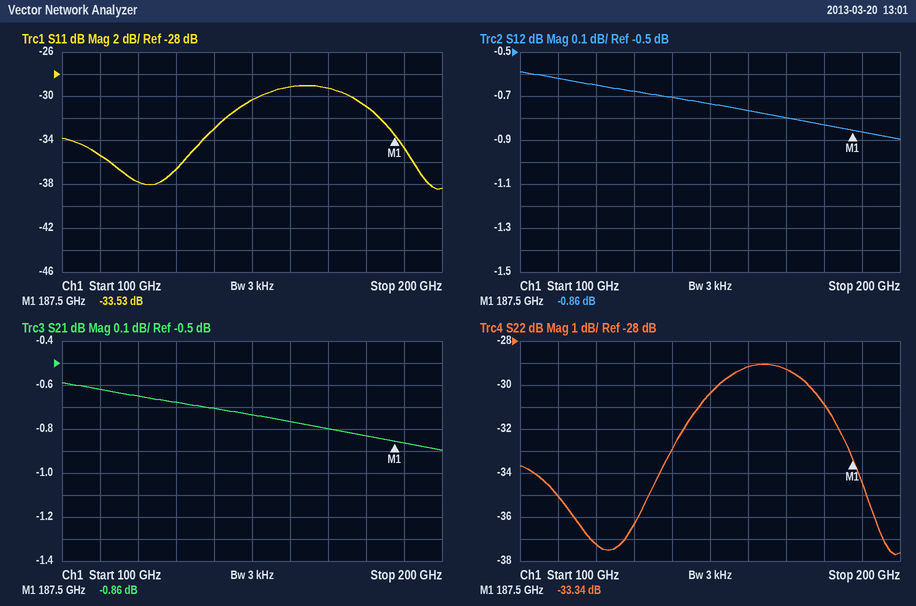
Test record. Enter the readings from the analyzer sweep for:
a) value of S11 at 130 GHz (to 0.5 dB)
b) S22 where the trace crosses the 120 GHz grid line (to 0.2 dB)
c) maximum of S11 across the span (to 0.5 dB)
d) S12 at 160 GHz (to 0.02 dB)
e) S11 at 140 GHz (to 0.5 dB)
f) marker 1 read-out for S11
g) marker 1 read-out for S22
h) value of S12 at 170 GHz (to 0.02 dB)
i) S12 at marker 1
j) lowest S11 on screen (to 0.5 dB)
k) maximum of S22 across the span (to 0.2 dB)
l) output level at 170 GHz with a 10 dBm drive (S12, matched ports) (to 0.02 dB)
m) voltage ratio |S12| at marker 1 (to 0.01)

-36.5 dB
-37.2 dB
-29.0 dB
-0.76 dB
-33.0 dB
-33.53 dB
-33.34 dB
-0.80 dB
-0.86 dB
-38.5 dB
-29.0 dB
9.20 dBm
0.91
